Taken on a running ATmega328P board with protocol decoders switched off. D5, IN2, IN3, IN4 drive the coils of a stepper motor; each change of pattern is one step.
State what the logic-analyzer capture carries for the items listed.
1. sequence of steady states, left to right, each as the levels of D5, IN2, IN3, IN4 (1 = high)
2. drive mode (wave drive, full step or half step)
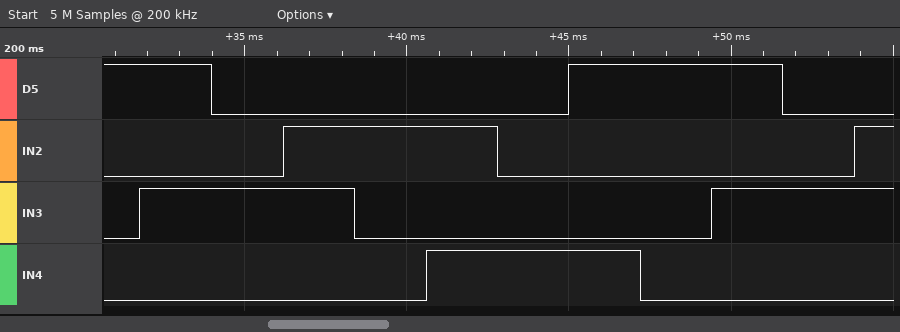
1000 1010 0010 0110 0100 0101 0001 1001 1000 1010 0010 0110
half step
